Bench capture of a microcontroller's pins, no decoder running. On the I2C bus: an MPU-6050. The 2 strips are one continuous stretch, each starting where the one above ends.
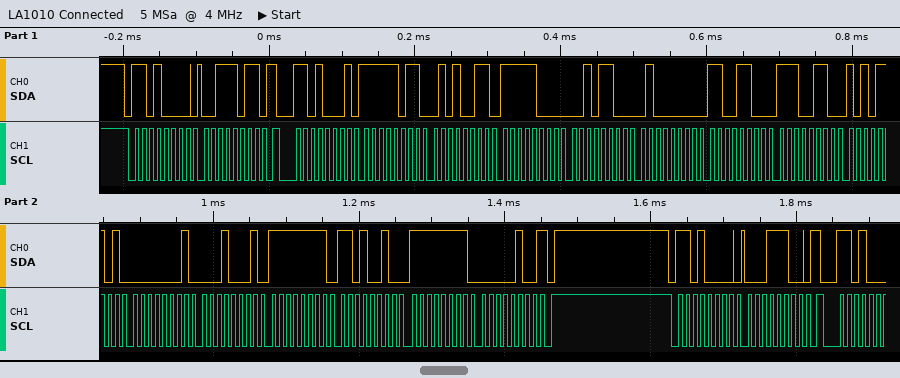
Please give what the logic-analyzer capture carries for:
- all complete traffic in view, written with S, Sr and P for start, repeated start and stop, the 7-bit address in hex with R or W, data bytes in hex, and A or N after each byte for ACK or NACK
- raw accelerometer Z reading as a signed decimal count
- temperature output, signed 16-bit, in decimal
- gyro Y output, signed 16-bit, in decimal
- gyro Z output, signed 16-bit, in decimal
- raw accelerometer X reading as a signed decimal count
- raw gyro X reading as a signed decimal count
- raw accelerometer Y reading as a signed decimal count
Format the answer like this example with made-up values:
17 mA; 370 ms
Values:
S 68W A 3B A Sr 68R A FB A 53 A F8 A 2C A 40 A CC A E6 A AD A 01 A 11 A FF A D2 A FF A 04 N P S 68W A 1C A; 16588; -6483; -46; -252; -1197; 273; -2004
